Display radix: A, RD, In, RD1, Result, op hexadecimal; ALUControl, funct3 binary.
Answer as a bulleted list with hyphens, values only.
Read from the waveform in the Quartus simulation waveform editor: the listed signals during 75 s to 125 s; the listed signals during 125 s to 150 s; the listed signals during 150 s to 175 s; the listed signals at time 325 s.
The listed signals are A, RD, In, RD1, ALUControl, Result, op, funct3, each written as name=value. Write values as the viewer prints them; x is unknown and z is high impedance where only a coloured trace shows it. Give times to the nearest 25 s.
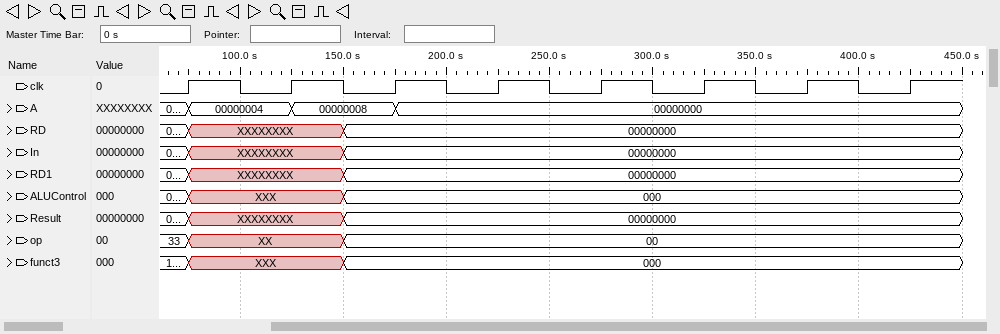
- A=00000004, RD=XXXXXXXX, In=XXXXXXXX, RD1=XXXXXXXX, ALUControl=XXX, Result=XXXXXXXX, op=XX, funct3=XXX
- A=00000008, RD=XXXXXXXX, In=XXXXXXXX, RD1=XXXXXXXX, ALUControl=XXX, Result=XXXXXXXX, op=XX, funct3=XXX
- A=00000008, RD=00000000, In=00000000, RD1=00000000, ALUControl=000, Result=00000000, op=00, funct3=000
- A=00000000, RD=00000000, In=00000000, RD1=00000000, ALUControl=000, Result=00000000, op=00, funct3=000
